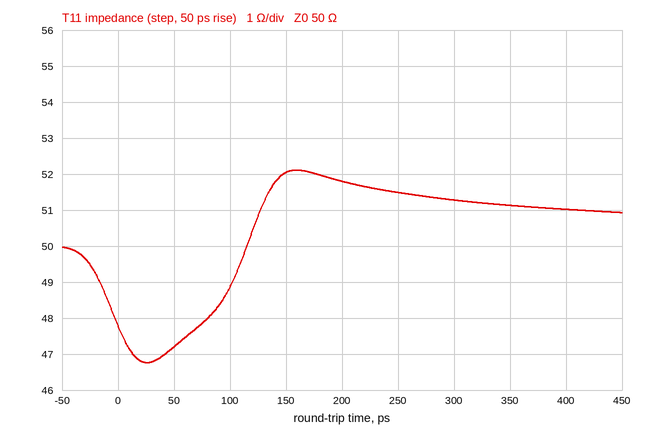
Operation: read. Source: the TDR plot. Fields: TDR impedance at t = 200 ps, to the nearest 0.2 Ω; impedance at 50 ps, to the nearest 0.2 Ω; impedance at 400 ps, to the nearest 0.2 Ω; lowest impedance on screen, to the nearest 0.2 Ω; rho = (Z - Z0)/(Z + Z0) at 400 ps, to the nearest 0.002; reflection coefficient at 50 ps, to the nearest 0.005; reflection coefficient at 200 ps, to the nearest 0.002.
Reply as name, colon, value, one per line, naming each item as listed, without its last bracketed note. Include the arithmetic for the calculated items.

TDR impedance at t = 200 ps, to the nearest 0.2 Ω: 51.8 Ω
impedance at 50 ps, to the nearest 0.2 Ω: 47.2 Ω
impedance at 400 ps, to the nearest 0.2 Ω: 51.0 Ω
lowest impedance on screen, to the nearest 0.2 Ω: 46.8 Ω
rho = (Z - Z0)/(Z + Z0) at 400 ps, to the nearest 0.002: (51 − 50)/(51 + 50) ≈ +0.010
reflection coefficient at 50 ps, to the nearest 0.005: (47.2 − 50)/(47.2 + 50) ≈ -0.0288, so -0.030 to the nearest 0.005
reflection coefficient at 200 ps, to the nearest 0.002: (51.8 − 50)/(51.8 + 50) ≈ +0.018
